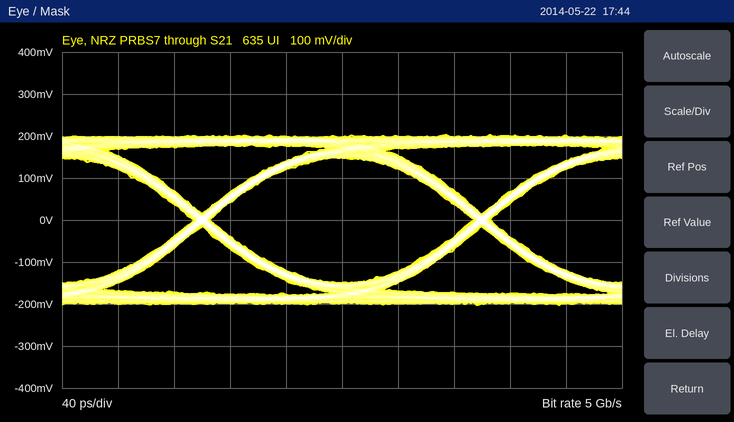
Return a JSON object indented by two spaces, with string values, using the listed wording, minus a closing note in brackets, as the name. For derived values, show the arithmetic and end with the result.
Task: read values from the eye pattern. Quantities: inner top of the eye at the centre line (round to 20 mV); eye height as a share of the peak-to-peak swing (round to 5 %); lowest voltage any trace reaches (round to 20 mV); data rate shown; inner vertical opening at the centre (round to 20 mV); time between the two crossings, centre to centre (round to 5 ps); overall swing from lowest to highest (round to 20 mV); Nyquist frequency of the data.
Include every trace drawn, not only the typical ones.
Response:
{
  "inner top of the eye at the centre line": "140 mV",
  "eye height as a share of the peak-to-peak swing": "300 mV / 400 mV ≈ 75 %",
  "lowest voltage any trace reaches": "-200 mV",
  "data rate shown": "5 Gb/s",
  "inner vertical opening at the centre": "300 mV",
  "time between the two crossings, centre to centre": "200 ps",
  "overall swing from lowest to highest": "400 mV",
  "Nyquist frequency of the data": "2.5 GHz"
}
